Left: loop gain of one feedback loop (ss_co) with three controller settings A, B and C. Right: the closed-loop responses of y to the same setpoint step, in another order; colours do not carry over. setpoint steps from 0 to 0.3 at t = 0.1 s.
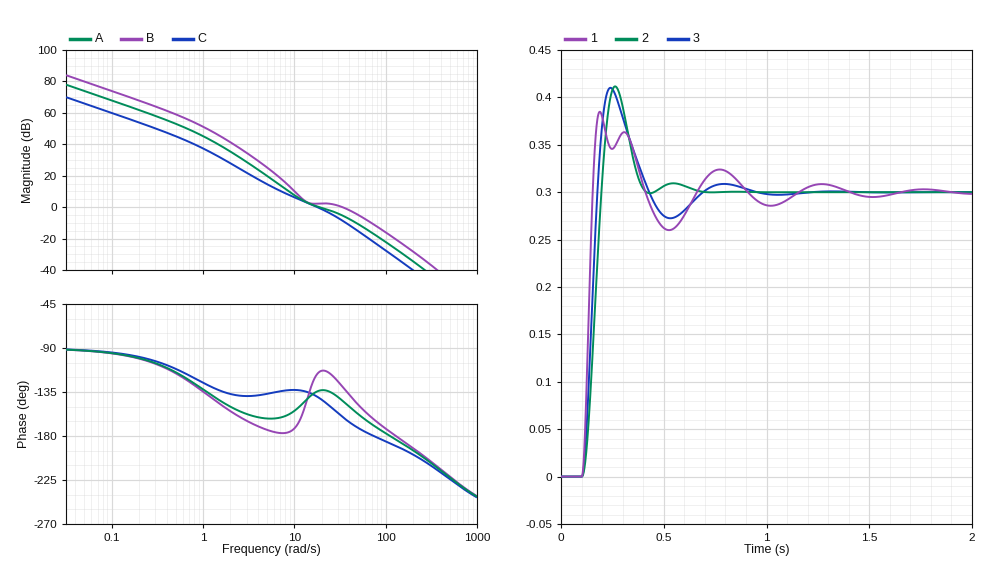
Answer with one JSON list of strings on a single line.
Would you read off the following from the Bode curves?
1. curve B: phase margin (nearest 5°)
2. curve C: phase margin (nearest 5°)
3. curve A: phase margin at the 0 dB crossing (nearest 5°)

["50°", "40°", "45°"]
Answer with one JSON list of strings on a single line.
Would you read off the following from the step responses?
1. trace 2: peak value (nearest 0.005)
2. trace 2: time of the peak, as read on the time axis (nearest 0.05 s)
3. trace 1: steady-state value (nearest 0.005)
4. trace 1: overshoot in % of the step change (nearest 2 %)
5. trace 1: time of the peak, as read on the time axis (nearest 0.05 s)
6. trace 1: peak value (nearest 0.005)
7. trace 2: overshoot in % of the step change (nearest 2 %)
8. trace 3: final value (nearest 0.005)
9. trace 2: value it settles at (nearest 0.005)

["0.410", "0.25 s", "0.300", "28 %", "0.20 s", "0.385", "38 %", "0.300", "0.300"]
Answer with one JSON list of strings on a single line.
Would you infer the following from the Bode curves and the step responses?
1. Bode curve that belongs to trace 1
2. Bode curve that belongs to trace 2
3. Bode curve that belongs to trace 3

["B", "C", "A"]
